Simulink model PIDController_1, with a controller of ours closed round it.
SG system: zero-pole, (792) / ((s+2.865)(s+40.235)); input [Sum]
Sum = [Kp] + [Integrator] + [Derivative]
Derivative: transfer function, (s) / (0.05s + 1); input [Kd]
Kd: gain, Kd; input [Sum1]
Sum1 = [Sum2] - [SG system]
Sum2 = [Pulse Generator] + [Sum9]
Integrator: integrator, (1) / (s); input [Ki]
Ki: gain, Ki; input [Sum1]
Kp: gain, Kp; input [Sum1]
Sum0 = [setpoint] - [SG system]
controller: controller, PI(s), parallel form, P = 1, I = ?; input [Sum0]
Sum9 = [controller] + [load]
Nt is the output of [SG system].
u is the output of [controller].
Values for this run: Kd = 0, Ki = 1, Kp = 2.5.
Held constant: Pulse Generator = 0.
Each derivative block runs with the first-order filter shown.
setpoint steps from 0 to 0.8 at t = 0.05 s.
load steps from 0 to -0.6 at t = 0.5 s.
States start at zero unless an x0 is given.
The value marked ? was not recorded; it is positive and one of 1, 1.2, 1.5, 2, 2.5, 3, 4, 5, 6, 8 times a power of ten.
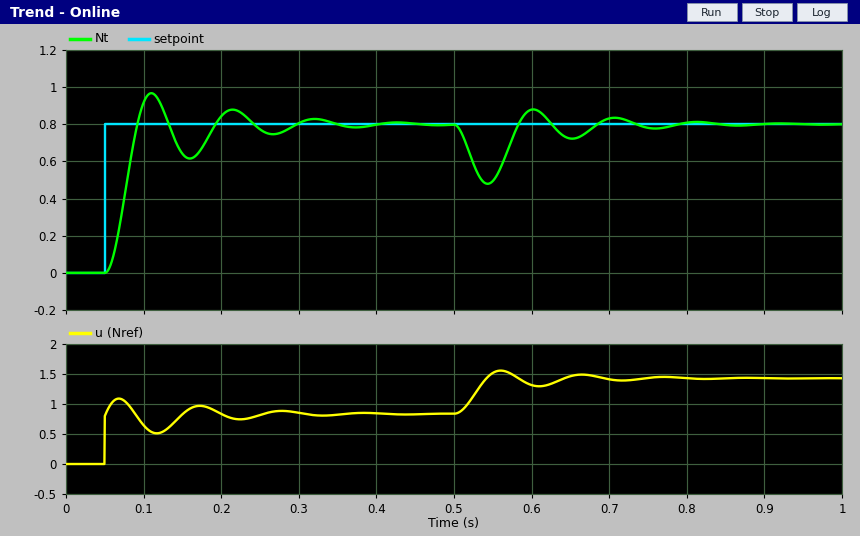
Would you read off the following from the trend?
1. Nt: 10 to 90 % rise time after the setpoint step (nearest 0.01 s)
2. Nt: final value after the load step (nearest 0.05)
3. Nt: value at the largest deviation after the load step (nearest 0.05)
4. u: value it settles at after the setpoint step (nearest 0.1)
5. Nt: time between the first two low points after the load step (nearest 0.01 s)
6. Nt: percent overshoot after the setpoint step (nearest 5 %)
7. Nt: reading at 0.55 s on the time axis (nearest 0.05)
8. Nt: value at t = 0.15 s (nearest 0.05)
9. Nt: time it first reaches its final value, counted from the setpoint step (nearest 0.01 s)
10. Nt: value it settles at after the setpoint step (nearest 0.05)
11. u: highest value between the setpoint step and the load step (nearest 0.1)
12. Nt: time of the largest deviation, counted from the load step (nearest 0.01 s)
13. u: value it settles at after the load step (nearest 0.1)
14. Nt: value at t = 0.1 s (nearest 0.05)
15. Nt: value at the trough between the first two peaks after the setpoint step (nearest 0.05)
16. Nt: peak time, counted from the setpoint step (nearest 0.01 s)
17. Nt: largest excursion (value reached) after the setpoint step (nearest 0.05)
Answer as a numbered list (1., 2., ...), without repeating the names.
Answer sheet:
1. 0.03 s
2. 0.80
3. 0.50
4. 0.8
5. 0.11 s
6. 20 %
7. 0.50
8. 0.65
9. 0.04 s
10. 0.80
11. 1.1
12. 0.04 s
13. 1.4
14. 0.90
15. 0.60
16. 0.06 s
17. 0.95
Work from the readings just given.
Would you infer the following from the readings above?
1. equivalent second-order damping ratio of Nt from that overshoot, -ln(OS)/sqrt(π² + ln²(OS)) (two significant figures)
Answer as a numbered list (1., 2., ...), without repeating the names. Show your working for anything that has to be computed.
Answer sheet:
1. ln(0.2) = -1.609; 1.609 / sqrt(9.870 + 2.590) = 0.46
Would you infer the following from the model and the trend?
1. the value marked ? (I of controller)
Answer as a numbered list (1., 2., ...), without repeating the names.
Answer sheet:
1. 40
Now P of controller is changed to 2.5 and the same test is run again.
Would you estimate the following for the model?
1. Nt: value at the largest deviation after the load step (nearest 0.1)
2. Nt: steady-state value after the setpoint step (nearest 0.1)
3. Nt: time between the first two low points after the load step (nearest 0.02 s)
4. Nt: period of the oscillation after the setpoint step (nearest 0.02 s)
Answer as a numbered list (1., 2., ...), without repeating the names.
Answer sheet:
1. 0.6
2. 0.8
3. 0.08 s
4. 0.08 s
